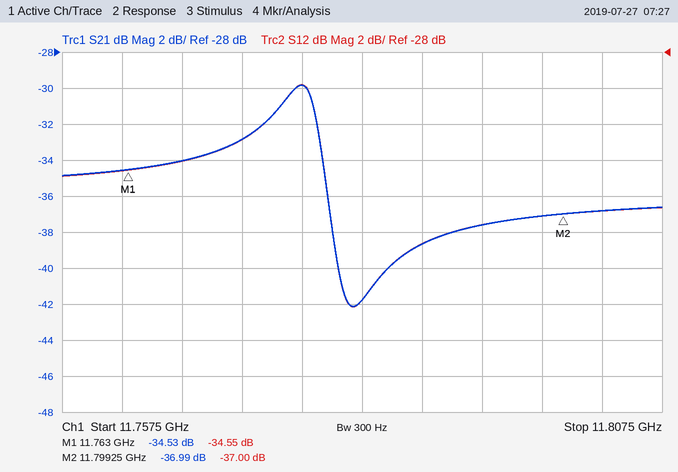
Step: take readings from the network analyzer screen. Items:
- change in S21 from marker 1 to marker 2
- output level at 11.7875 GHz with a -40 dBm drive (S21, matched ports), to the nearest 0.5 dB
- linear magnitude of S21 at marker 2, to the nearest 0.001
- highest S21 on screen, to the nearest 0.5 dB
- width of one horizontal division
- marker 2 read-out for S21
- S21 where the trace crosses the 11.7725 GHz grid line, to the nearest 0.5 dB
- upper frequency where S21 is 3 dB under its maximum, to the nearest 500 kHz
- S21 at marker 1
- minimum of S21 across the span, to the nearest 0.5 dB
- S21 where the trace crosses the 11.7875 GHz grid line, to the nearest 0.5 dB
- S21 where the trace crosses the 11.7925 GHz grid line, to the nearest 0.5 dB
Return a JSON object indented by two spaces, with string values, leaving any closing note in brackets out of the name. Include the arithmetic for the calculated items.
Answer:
{
  "change in S21 from marker 1 to marker 2": "-36.99 − (-34.53) = -2.46 dB",
  "output level at 11.7875 GHz with a -40 dBm drive (S21, matched ports), to the nearest 0.5 dB": "-40 dBm + (-38.5 dB) = -78.5 dBm",
  "linear magnitude of S21 at marker 2, to the nearest 0.001": "10^(-36.99/20) ≈ 0.014",
  "highest S21 on screen, to the nearest 0.5 dB": "-30.0 dB",
  "width of one horizontal division": "5 MHz",
  "marker 2 read-out for S21": "-36.99 dB",
  "S21 where the trace crosses the 11.7725 GHz grid line, to the nearest 0.5 dB": "-33.0 dB",
  "upper frequency where S21 is 3 dB under its maximum, to the nearest 500 kHz": "11.7790 GHz",
  "S21 at marker 1": "-34.53 dB",
  "minimum of S21 across the span, to the nearest 0.5 dB": "-42.0 dB",
  "S21 where the trace crosses the 11.7875 GHz grid line, to the nearest 0.5 dB": "-38.5 dB",
  "S21 where the trace crosses the 11.7925 GHz grid line, to the nearest 0.5 dB": "-37.5 dB"
}
